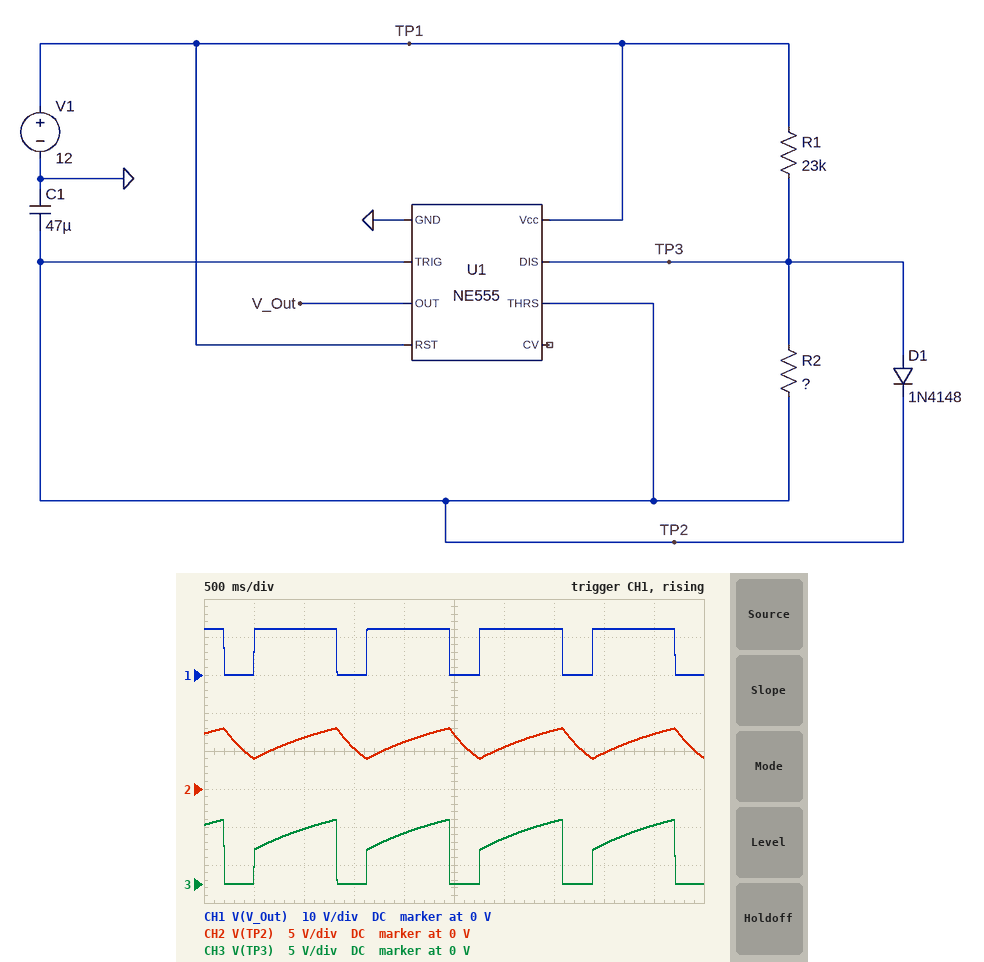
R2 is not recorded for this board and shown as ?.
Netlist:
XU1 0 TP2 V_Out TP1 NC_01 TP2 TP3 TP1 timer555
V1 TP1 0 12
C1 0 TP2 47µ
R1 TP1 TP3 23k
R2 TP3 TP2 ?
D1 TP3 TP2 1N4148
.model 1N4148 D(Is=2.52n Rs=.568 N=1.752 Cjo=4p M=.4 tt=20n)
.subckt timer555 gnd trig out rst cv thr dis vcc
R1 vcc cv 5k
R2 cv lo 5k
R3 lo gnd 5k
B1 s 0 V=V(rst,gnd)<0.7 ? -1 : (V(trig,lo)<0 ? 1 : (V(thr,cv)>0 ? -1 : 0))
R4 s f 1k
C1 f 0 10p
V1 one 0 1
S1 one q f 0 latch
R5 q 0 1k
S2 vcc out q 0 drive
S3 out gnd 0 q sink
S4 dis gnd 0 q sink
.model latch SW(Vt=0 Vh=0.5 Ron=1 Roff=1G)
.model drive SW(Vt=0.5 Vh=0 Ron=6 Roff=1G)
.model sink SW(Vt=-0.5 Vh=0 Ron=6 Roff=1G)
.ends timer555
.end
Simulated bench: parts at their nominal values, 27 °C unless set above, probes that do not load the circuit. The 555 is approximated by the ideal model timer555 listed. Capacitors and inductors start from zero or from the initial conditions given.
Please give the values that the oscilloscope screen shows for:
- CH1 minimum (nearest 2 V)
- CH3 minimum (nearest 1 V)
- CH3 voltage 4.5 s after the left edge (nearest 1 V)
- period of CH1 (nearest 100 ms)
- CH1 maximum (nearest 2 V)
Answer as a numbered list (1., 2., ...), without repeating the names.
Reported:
1. 0 V
2. 0 V
3. 8 V
4. 1.1 s
5. 12 V
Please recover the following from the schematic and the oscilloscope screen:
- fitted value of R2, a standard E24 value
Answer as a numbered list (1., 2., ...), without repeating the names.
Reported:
1. 9.1 kΩ
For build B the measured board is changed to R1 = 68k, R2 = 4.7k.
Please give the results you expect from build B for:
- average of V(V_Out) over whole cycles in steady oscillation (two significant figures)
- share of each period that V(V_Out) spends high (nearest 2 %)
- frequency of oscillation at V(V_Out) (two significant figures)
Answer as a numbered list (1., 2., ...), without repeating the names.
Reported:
1. 11 V
2. 94 %
3. 400 mHz
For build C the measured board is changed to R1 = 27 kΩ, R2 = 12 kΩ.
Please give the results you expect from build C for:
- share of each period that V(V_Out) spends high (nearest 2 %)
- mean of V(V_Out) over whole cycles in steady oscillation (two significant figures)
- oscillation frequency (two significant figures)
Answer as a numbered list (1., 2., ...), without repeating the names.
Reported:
1. 72 %
2. 8.5 V
3. 740 mHz
